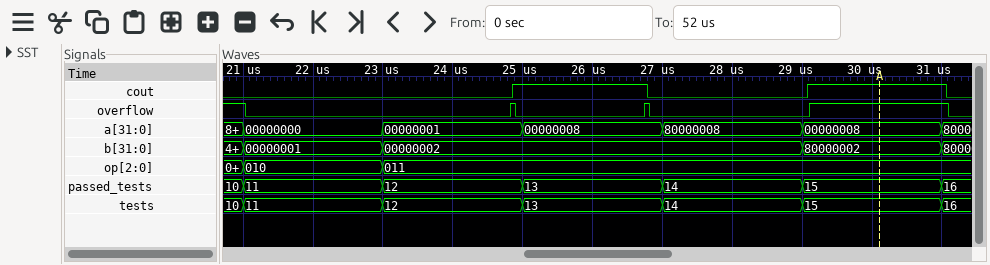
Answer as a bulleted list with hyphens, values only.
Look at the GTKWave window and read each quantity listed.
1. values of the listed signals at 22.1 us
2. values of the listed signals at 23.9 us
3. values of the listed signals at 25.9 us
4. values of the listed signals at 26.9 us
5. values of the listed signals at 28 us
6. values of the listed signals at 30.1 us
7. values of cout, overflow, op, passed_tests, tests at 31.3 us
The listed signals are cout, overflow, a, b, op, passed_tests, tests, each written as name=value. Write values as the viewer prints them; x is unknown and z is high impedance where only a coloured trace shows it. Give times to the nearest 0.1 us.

- cout=0, overflow=0, a=00000000, b=00000001, op=010, passed_tests=11, tests=11
- cout=0, overflow=0, a=00000001, b=00000002, op=011, passed_tests=12, tests=12
- cout=1, overflow=0, a=00000008, b=00000002, op=011, passed_tests=13, tests=13
- cout=0, overflow=0, a=00000008, b=00000002, op=011, passed_tests=13, tests=13
- cout=0, overflow=0, a=80000008, b=00000002, op=011, passed_tests=14, tests=14
- cout=1, overflow=1, a=00000008, b=80000002, op=011, passed_tests=15, tests=15
- cout=0, overflow=0, op=011, passed_tests=16, tests=16
